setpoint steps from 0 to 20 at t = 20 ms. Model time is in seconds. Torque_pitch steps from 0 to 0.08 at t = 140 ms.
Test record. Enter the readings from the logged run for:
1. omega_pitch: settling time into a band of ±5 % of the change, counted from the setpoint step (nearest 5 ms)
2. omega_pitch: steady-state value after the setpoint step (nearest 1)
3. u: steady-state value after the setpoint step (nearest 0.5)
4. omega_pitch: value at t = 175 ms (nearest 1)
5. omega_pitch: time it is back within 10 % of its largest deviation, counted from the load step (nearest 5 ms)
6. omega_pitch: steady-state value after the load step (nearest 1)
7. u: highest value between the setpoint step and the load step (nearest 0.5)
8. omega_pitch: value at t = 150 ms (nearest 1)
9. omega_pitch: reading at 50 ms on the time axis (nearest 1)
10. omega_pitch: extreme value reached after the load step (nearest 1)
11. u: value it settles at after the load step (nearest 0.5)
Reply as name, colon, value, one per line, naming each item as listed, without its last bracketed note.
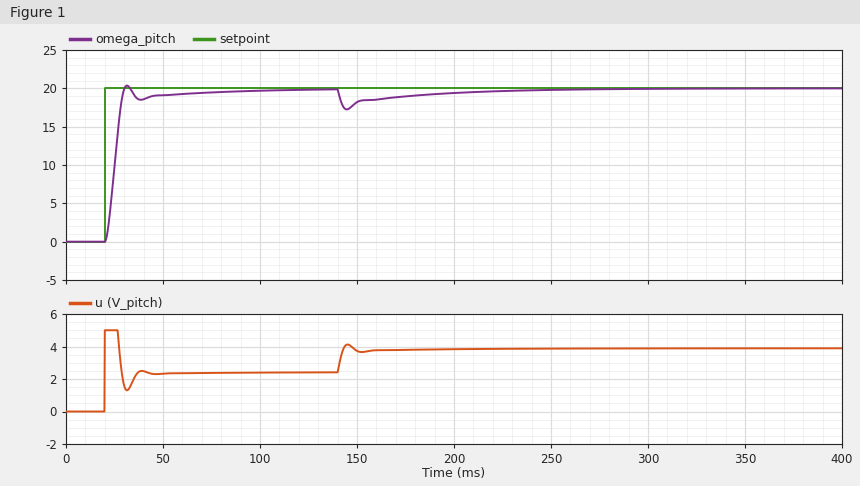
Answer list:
omega_pitch: settling time into a band of ±5 % of the change, counted from the setpoint step: 25 ms
omega_pitch: steady-state value after the setpoint step: 20
u: steady-state value after the setpoint step: 2.5
omega_pitch: value at t = 175 ms: 19
omega_pitch: time it is back within 10 % of its largest deviation, counted from the load step: 100 ms
omega_pitch: steady-state value after the load step: 20
u: highest value between the setpoint step and the load step: 5.0
omega_pitch: value at t = 150 ms: 18
omega_pitch: reading at 50 ms on the time axis: 19
omega_pitch: extreme value reached after the load step: 17
u: value it settles at after the load step: 4.0
